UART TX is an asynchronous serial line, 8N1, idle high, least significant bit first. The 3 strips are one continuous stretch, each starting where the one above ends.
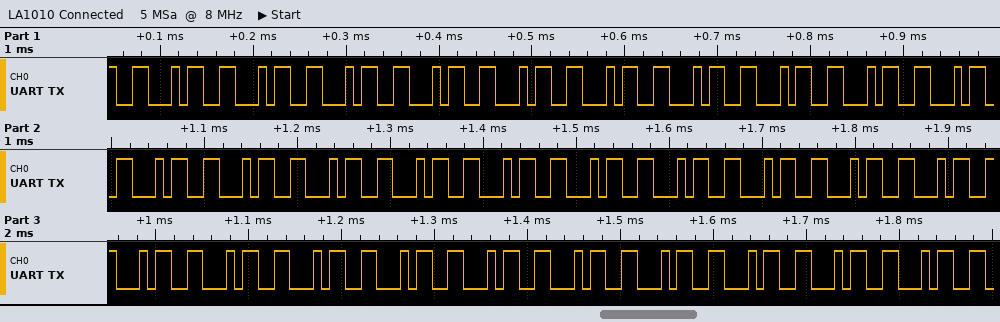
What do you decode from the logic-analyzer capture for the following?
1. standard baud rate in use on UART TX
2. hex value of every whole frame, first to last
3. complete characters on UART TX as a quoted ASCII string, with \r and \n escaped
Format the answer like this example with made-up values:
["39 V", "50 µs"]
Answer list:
["115200 baud", "46 46 46 46 46 46 46 46 46 46 46 46 46 46 46 46 46 46 46 46 46 46 46 46 46 46 46 46 46 46", "\"FFFFFFFFFFFFFFFFFFFFFFFFFFFFFF\""]
